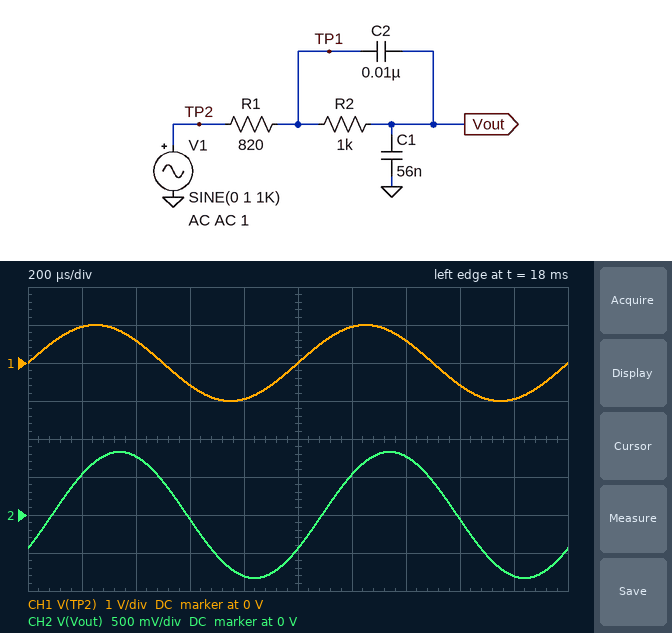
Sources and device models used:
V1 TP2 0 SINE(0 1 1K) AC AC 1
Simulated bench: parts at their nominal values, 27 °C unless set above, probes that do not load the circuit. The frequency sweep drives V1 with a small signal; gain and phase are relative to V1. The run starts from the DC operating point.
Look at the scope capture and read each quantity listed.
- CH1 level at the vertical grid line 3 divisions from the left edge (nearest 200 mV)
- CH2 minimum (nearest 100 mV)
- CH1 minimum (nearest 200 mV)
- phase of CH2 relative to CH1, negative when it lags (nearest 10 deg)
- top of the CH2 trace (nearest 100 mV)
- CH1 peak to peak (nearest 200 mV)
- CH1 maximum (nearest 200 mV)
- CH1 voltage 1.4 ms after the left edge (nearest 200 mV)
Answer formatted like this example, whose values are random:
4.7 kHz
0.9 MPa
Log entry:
-600 mV
-800 mV
-1.0 V
-30 deg
800 mV
2.0 V
1.0 V
600 mV
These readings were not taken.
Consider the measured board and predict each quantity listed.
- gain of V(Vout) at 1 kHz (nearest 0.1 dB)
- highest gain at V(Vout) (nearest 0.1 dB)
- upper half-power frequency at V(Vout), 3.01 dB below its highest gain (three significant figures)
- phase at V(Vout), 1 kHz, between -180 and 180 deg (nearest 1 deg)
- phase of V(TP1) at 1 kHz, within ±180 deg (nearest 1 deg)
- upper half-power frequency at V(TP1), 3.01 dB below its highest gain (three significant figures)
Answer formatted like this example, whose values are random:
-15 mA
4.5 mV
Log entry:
-1.6 dB
0 dB
1.49 kHz
-32 deg
-13 deg
2.92 kHz
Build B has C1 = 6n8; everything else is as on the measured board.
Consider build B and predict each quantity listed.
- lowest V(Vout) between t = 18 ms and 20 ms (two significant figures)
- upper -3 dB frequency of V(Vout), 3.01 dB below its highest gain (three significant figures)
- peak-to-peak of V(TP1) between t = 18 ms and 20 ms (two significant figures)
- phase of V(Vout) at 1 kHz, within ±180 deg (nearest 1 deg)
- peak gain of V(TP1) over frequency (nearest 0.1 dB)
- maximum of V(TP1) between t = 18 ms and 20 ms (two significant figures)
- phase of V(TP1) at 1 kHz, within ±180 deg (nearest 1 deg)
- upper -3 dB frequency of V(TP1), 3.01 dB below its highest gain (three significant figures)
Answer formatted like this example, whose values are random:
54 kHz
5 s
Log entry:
-990 mV
11.1 kHz
2.0 V
-4 deg
0 dB
1.0 V
-2 deg
39.5 kHz
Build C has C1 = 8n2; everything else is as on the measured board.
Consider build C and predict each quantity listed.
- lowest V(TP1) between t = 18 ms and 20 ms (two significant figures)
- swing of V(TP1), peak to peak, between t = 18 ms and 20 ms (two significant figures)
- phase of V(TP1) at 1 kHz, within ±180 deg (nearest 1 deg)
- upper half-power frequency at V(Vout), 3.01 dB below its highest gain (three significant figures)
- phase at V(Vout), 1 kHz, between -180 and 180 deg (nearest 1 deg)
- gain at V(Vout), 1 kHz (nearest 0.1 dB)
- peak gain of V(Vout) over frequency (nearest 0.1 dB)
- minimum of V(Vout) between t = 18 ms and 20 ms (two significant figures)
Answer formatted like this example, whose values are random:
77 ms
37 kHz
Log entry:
-1.0 V
2.0 V
-2 deg
9.16 kHz
-5 deg
-0.1 dB
0 dB
-990 mV
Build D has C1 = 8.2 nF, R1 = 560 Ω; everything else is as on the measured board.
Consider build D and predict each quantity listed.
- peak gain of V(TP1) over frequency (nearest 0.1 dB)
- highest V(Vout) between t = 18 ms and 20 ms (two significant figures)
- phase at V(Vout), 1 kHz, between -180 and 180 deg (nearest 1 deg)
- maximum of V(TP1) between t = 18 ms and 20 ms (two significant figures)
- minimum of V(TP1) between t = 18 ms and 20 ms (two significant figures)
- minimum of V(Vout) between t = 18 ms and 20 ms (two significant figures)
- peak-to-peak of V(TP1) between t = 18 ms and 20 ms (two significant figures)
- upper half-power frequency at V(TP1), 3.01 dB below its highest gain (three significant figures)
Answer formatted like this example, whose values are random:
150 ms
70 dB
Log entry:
0 dB
990 mV
-5 deg
1.0 V
-1.0 V
-990 mV
2.0 V
54.1 kHz
